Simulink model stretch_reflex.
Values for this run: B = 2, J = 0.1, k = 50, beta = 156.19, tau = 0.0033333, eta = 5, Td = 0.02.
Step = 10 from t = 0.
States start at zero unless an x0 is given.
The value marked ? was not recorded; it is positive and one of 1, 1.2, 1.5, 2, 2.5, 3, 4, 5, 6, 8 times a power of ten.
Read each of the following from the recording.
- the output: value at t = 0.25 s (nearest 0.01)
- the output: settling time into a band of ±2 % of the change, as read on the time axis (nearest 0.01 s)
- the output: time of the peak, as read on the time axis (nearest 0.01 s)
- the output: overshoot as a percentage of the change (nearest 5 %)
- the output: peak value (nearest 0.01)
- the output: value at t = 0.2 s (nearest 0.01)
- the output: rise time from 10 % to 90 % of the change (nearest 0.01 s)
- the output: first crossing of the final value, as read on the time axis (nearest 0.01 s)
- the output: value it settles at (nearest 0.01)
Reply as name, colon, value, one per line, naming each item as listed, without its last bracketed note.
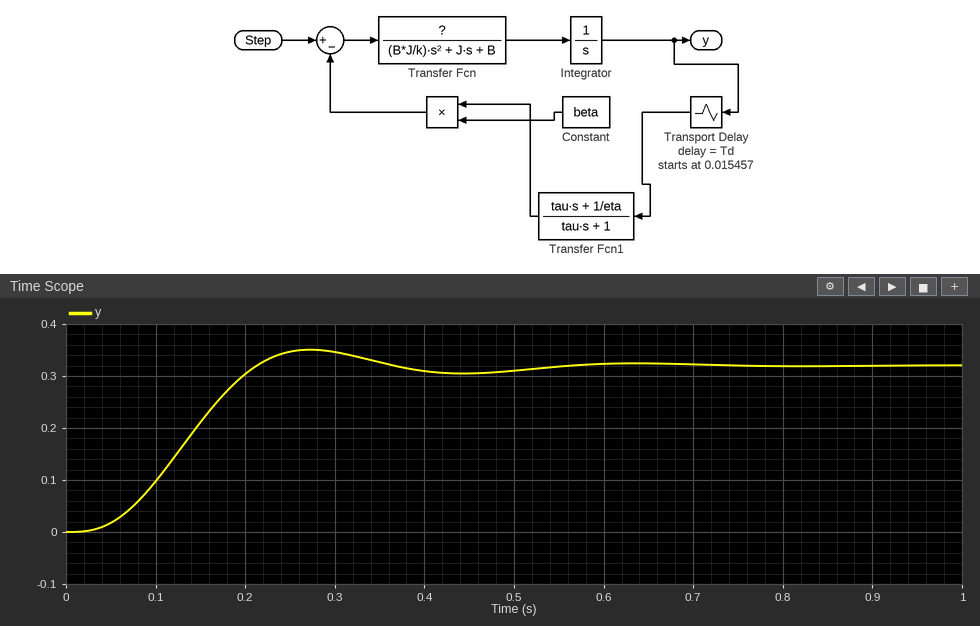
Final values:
the output: value at t = 0.25 s: 0.35
the output: settling time into a band of ±2 % of the change, as read on the time axis: 0.52 s
the output: time of the peak, as read on the time axis: 0.27 s
the output: overshoot as a percentage of the change: 10 %
the output: peak value: 0.35
the output: value at t = 0.2 s: 0.30
the output: rise time from 10 % to 90 % of the change: 0.13 s
the output: first crossing of the final value, as read on the time axis: 0.21 s
the output: value it settles at: 0.32
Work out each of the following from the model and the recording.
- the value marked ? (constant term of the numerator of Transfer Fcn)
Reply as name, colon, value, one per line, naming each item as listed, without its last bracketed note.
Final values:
the value marked ?: 0.5
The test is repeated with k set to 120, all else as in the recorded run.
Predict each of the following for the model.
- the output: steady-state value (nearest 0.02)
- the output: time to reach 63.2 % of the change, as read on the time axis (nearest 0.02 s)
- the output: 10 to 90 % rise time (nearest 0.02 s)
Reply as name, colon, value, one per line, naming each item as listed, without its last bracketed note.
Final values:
the output: steady-state value: 0.32
the output: time to reach 63.2 % of the change, as read on the time axis: 0.14 s
the output: 10 to 90 % rise time: 0.16 s
